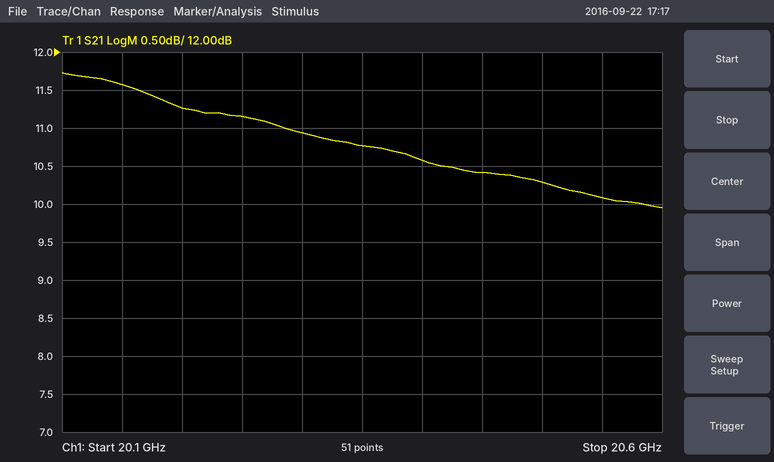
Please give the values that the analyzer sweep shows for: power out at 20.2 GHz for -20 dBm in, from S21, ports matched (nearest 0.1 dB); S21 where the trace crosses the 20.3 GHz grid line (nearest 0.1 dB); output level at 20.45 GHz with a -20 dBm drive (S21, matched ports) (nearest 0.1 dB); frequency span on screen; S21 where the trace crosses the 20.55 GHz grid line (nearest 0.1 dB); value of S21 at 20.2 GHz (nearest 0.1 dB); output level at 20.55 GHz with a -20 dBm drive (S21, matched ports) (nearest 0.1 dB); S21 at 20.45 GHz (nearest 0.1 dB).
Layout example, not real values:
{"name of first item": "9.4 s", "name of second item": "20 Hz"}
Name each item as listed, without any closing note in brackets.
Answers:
{"power out at 20.2 GHz for -20 dBm in, from S21, ports matched": "-8.7 dBm", "S21 where the trace crosses the 20.3 GHz grid line": "10.9 dB", "output level at 20.45 GHz with a -20 dBm drive (S21, matched ports)": "-9.6 dBm", "frequency span on screen": "500 MHz", "S21 where the trace crosses the 20.55 GHz grid line": "10.1 dB", "value of S21 at 20.2 GHz": "11.3 dB", "output level at 20.55 GHz with a -20 dBm drive (S21, matched ports)": "-9.9 dBm", "S21 at 20.45 GHz": "10.4 dB"}
